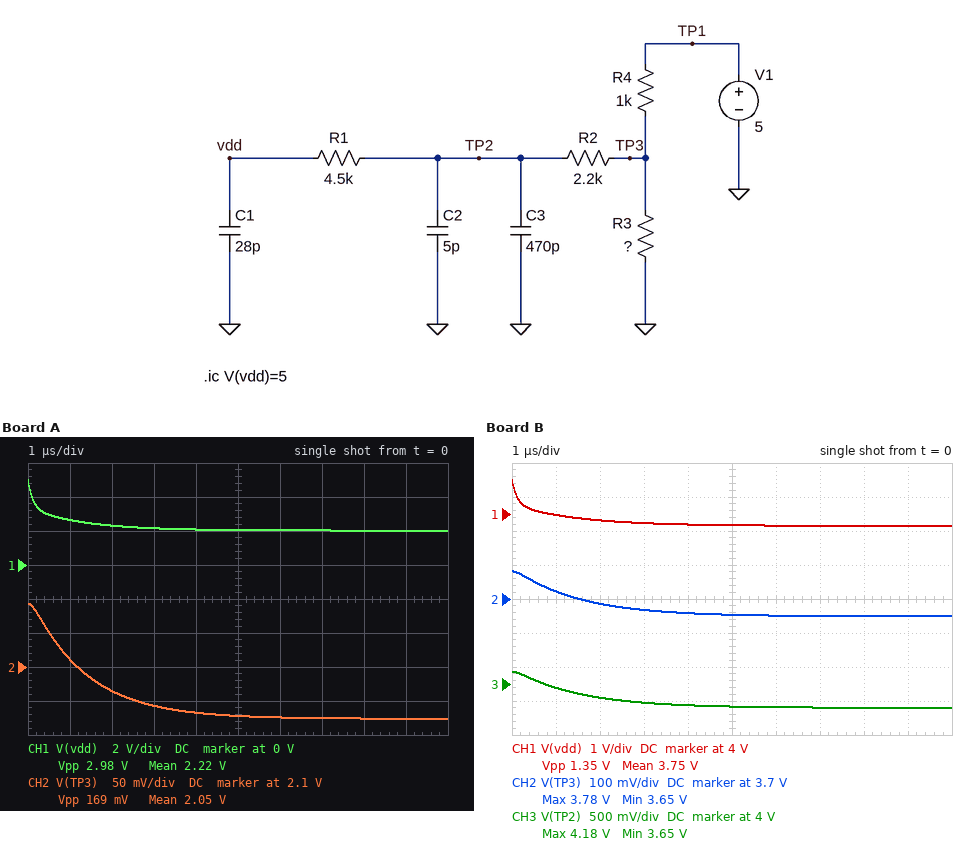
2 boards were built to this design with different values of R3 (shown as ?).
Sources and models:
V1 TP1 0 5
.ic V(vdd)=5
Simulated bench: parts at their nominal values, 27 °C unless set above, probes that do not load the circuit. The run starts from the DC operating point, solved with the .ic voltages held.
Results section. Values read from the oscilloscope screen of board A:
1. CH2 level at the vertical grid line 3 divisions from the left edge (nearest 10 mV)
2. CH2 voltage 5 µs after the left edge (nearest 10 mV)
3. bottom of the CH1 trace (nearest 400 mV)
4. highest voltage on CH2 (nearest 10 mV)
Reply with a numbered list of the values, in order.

1. 2.04 V
2. 2.03 V
3. 2.0 V
4. 2.19 V
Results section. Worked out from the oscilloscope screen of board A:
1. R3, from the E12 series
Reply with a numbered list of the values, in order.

1. 680 Ω
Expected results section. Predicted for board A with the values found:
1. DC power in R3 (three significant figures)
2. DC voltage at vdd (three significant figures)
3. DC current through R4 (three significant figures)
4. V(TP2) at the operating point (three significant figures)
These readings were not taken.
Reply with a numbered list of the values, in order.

1. 6.02 mW
2. 2.02 V
3. 2.98 mA
4. 2.02 V
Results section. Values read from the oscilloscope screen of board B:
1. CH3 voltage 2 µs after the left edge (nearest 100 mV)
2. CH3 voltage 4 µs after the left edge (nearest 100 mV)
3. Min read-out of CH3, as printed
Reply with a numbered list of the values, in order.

1. 3.8 V
2. 3.7 V
3. 3.65 V
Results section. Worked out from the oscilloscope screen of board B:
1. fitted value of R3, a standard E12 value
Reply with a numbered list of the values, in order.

1. 2.7 kΩ
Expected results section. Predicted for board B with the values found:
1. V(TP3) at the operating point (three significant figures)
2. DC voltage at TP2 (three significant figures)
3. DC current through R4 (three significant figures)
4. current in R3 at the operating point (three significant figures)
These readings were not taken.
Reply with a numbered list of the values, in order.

1. 3.65 V
2. 3.65 V
3. 1.35 mA
4. 1.35 mA
